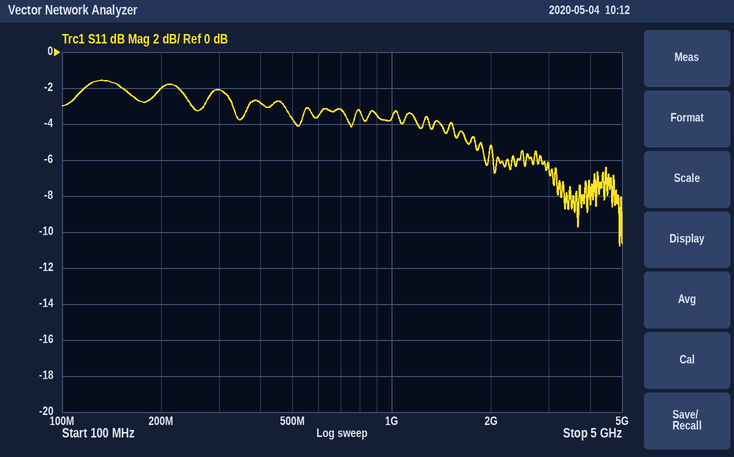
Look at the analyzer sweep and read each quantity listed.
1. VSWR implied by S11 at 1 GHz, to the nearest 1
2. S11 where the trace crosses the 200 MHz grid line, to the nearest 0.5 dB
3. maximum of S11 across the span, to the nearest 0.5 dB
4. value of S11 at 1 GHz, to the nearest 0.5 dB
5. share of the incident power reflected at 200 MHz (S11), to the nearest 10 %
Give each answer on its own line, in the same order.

5
-2.0 dB
-1.5 dB
-3.5 dB
60 %
